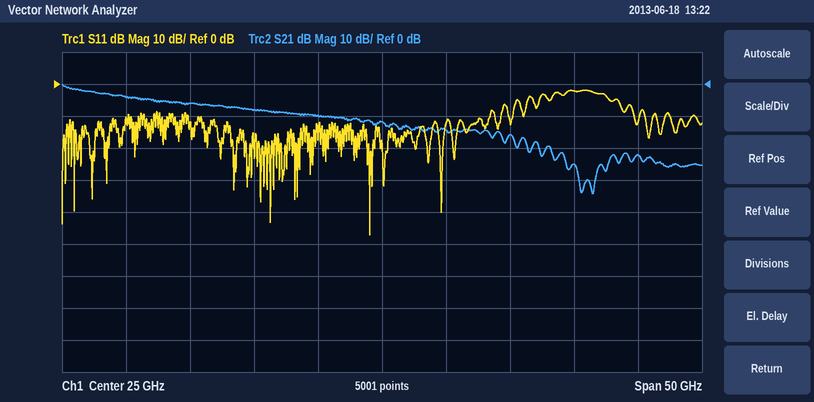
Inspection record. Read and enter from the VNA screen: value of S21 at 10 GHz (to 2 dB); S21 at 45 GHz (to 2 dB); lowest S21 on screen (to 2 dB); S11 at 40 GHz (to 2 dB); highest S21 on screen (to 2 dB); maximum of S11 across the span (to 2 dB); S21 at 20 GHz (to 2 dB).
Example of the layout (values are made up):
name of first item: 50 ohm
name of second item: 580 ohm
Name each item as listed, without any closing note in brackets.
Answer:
value of S21 at 10 GHz: -6 dB
S21 at 45 GHz: -22 dB
lowest S21 on screen: -34 dB
S11 at 40 GHz: -2 dB
highest S21 on screen: 0 dB
maximum of S11 across the span: -2 dB
S21 at 20 GHz: -10 dB
